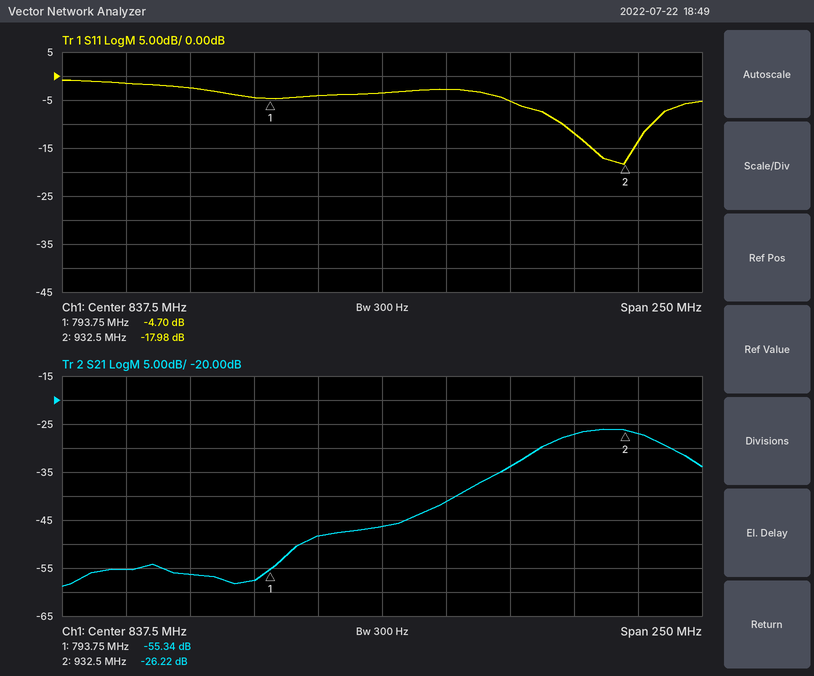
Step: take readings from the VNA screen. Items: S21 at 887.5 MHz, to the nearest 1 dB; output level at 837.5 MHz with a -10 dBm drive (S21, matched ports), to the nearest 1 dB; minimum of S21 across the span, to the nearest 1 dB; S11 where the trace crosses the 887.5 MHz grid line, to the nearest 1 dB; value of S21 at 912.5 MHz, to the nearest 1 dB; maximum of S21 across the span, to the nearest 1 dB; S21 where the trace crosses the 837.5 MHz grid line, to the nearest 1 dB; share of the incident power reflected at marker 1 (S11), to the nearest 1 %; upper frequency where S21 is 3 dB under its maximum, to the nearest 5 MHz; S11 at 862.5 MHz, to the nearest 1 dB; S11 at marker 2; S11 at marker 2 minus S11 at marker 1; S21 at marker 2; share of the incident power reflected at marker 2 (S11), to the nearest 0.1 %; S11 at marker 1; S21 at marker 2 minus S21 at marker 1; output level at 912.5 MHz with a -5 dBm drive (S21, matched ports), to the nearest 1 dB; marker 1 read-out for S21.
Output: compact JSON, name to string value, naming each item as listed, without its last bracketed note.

{"S21 at 887.5 MHz, to the nearest 1 dB": "-34 dB", "output level at 837.5 MHz with a -10 dBm drive (S21, matched ports), to the nearest 1 dB": "-56 dBm", "minimum of S21 across the span, to the nearest 1 dB": "-59 dB", "S11 where the trace crosses the 887.5 MHz grid line, to the nearest 1 dB": "-5 dB", "value of S21 at 912.5 MHz, to the nearest 1 dB": "-27 dB", "maximum of S21 across the span, to the nearest 1 dB": "-26 dB", "S21 where the trace crosses the 837.5 MHz grid line, to the nearest 1 dB": "-46 dB", "share of the incident power reflected at marker 1 (S11), to the nearest 1 %": "34 %", "upper frequency where S21 is 3 dB under its maximum, to the nearest 5 MHz": "945 MHz", "S11 at 862.5 MHz, to the nearest 1 dB": "-3 dB", "S11 at marker 2": "-17.98 dB", "S11 at marker 2 minus S11 at marker 1": "-13.28 dB", "S21 at marker 2": "-26.22 dB", "share of the incident power reflected at marker 2 (S11), to the nearest 0.1 %": "1.6 %", "S11 at marker 1": "-4.70 dB", "S21 at marker 2 minus S21 at marker 1": "29.12 dB", "output level at 912.5 MHz with a -5 dBm drive (S21, matched ports), to the nearest 1 dB": "-32 dBm", "marker 1 read-out for S21": "-55.34 dB"}
